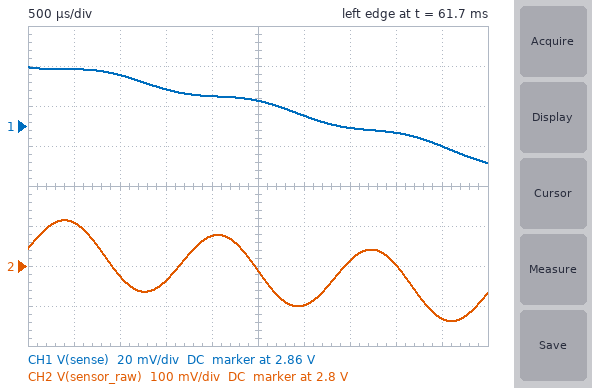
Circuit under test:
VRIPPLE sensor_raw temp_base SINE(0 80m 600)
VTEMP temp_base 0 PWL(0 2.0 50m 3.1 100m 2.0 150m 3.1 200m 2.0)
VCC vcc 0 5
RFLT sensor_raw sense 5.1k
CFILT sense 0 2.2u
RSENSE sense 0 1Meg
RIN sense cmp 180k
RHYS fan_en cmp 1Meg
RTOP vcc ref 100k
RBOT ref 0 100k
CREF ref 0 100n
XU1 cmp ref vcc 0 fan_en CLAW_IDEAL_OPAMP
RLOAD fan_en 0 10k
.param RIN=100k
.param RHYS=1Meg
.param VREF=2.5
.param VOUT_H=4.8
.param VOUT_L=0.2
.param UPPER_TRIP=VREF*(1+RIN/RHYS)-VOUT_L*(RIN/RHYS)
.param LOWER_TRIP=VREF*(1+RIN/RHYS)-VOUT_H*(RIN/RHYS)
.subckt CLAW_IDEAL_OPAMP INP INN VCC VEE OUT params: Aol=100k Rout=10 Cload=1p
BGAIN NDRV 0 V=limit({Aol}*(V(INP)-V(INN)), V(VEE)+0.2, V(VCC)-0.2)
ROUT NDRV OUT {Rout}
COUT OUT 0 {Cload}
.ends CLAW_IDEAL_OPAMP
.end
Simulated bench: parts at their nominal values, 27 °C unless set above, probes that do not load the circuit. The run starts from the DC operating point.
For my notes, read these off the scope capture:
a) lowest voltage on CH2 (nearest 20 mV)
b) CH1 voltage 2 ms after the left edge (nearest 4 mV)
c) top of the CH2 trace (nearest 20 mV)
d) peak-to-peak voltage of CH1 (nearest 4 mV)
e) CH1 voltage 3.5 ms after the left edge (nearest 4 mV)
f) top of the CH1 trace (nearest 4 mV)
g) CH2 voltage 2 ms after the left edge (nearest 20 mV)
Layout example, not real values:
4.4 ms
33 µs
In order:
2.66 V
2.876 V
2.92 V
48 mV
2.860 V
2.888 V
2.88 V
